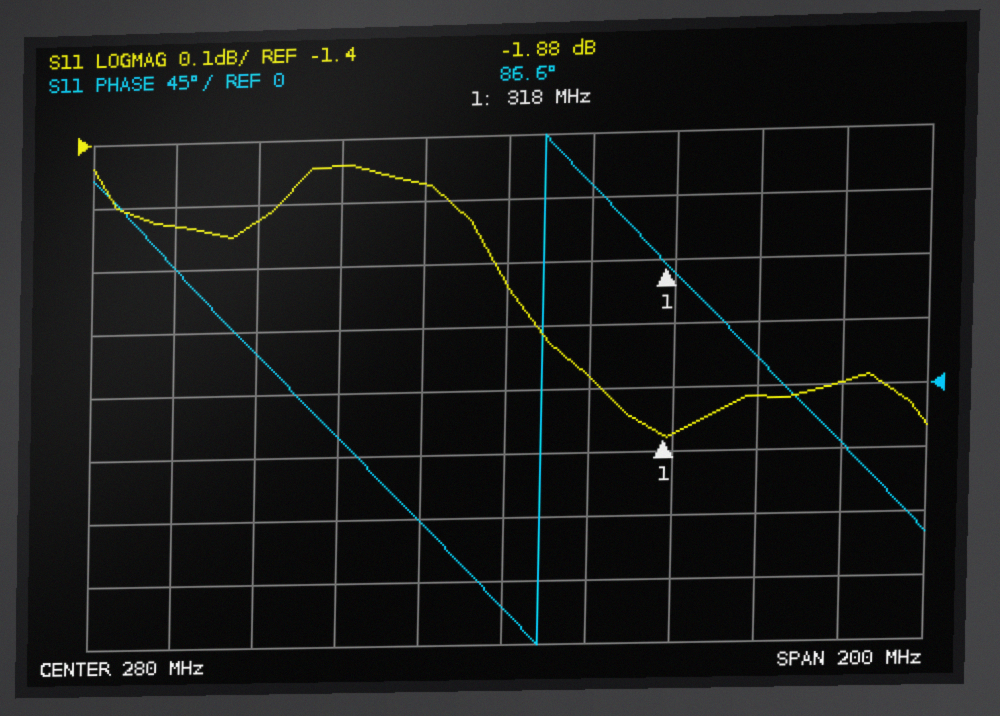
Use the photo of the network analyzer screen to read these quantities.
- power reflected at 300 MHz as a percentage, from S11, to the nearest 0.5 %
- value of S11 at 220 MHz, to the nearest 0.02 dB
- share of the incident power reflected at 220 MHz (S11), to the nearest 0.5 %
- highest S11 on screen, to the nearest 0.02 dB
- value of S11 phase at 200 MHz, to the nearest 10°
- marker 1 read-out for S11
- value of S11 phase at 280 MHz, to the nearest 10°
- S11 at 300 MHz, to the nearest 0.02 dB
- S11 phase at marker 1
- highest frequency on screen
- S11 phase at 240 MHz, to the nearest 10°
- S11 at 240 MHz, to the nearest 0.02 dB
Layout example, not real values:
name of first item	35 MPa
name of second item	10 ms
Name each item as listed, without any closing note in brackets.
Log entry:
power reflected at 300 MHz as a percentage, from S11, to the nearest 0.5 %	66.5 %
value of S11 at 220 MHz, to the nearest 0.02 dB	-1.52 dB
share of the incident power reflected at 220 MHz (S11), to the nearest 0.5 %	70.5 %
highest S11 on screen, to the nearest 0.02 dB	-1.44 dB
value of S11 phase at 200 MHz, to the nearest 10°	90°
marker 1 read-out for S11	-1.88 dB
value of S11 phase at 280 MHz, to the nearest 10°	-150°
S11 at 300 MHz, to the nearest 0.02 dB	-1.78 dB
S11 phase at marker 1	86.6°
highest frequency on screen	380 MHz
S11 phase at 240 MHz, to the nearest 10°	-30°
S11 at 240 MHz, to the nearest 0.02 dB	-1.44 dB
